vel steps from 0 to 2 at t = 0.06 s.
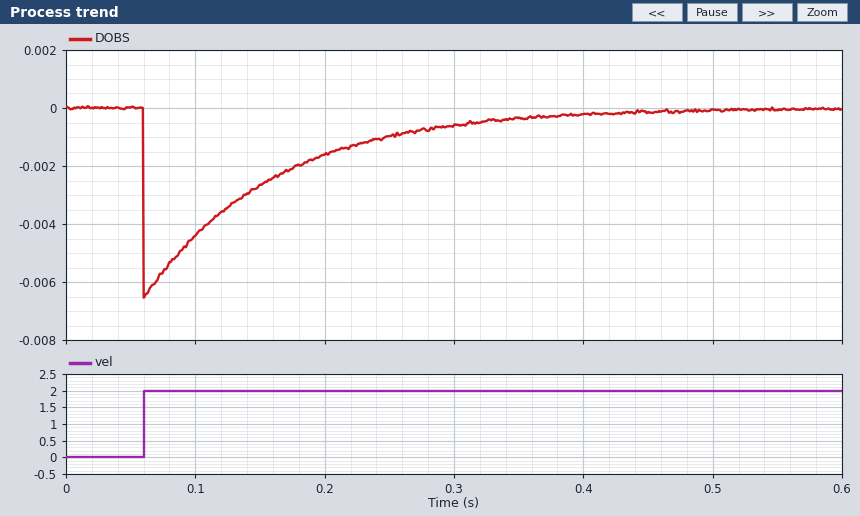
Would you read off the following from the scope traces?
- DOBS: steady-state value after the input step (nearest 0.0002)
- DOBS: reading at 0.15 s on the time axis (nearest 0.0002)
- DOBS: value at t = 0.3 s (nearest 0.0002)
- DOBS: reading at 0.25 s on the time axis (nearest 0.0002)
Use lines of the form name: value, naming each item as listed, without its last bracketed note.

DOBS: steady-state value after the input step: 0.0000
DOBS: reading at 0.15 s on the time axis: -0.0026
DOBS: value at t = 0.3 s: -0.0006
DOBS: reading at 0.25 s on the time axis: -0.0010
